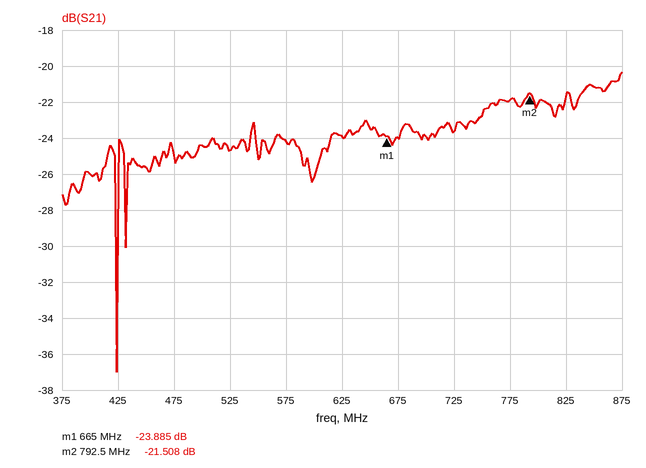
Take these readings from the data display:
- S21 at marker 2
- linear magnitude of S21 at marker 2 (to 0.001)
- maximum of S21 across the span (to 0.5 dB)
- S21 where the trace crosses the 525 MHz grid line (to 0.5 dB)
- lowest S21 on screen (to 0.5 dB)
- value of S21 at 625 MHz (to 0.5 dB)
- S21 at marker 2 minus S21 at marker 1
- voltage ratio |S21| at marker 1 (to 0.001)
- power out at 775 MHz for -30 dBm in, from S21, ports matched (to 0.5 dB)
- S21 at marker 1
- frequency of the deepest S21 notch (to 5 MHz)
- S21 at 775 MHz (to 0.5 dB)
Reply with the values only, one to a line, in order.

-21.508 dB
0.084
-20.5 dB
-24.5 dB
-37.0 dB
-24.0 dB
2.377 dB
0.064
-52.0 dBm
-23.885 dB
425 MHz
-22.0 dB
